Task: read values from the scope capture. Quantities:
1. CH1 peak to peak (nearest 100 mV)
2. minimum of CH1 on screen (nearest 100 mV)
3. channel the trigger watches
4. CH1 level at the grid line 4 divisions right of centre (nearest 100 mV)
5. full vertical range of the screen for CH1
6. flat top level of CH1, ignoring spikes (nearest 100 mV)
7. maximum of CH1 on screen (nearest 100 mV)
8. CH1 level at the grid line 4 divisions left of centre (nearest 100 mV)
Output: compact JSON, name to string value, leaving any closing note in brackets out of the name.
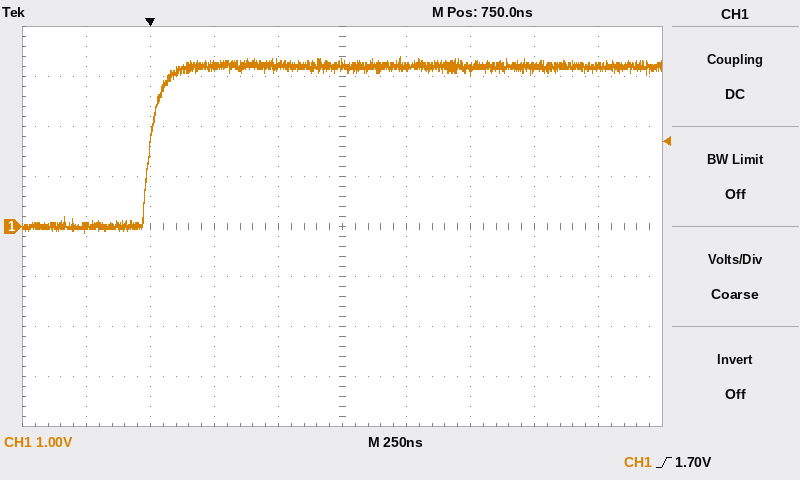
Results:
{"CH1 peak to peak": "3.5 V", "minimum of CH1 on screen": "-100 mV", "channel the trigger watches": "CH1", "CH1 level at the grid line 4 divisions right of centre": "3.2 V", "full vertical range of the screen for CH1": "8 V", "flat top level of CH1, ignoring spikes": "3.2 V", "maximum of CH1 on screen": "3.4 V", "CH1 level at the grid line 4 divisions left of centre": "0.0 V"}
